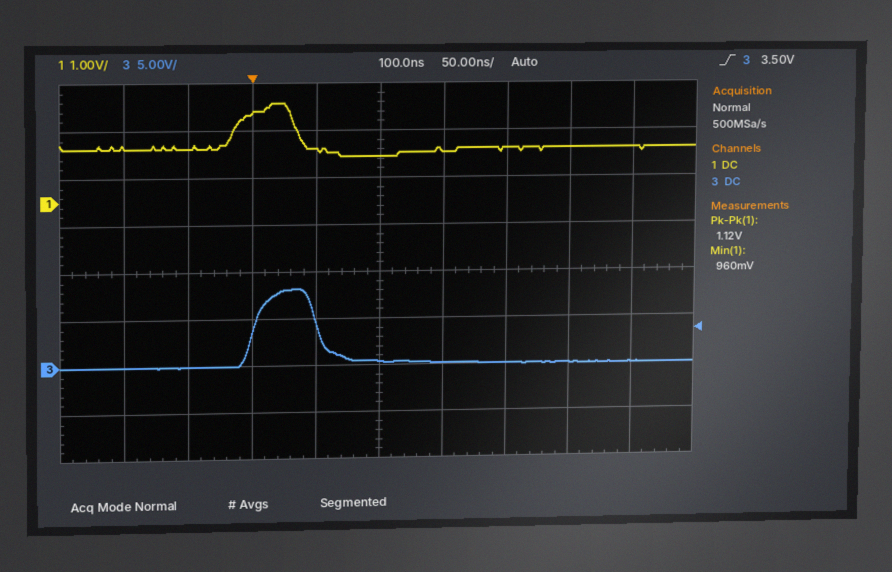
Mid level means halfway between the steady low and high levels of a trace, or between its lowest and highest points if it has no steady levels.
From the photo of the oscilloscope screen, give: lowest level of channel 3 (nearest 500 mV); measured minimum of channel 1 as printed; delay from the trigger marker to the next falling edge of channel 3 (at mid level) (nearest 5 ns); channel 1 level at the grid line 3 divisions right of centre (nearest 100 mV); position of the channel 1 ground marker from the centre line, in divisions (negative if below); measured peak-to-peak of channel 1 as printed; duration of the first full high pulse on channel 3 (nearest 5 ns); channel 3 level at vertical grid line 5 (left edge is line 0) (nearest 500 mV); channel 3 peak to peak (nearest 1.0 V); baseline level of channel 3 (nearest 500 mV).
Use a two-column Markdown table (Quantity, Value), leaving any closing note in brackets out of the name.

| Quantity | Value |
|---|---|
| lowest level of channel 3 | 0.0 V |
| measured minimum of channel 1 as printed | 960 mV |
| delay from the trigger marker to the next falling edge of channel 3 (at mid level) | 50 ns |
| channel 1 level at the grid line 3 divisions right of centre | 1.1 V |
| position of the channel 1 ground marker from the centre line, in divisions | +1.5 div |
| measured peak-to-peak of channel 1 as printed | 1.12 V |
| duration of the first full high pulse on channel 3 | 50 ns |
| channel 3 level at vertical grid line 5 (left edge is line 0) | 500 mV |
| channel 3 peak to peak | 8.0 V |
| baseline level of channel 3 | 0.0 V |
